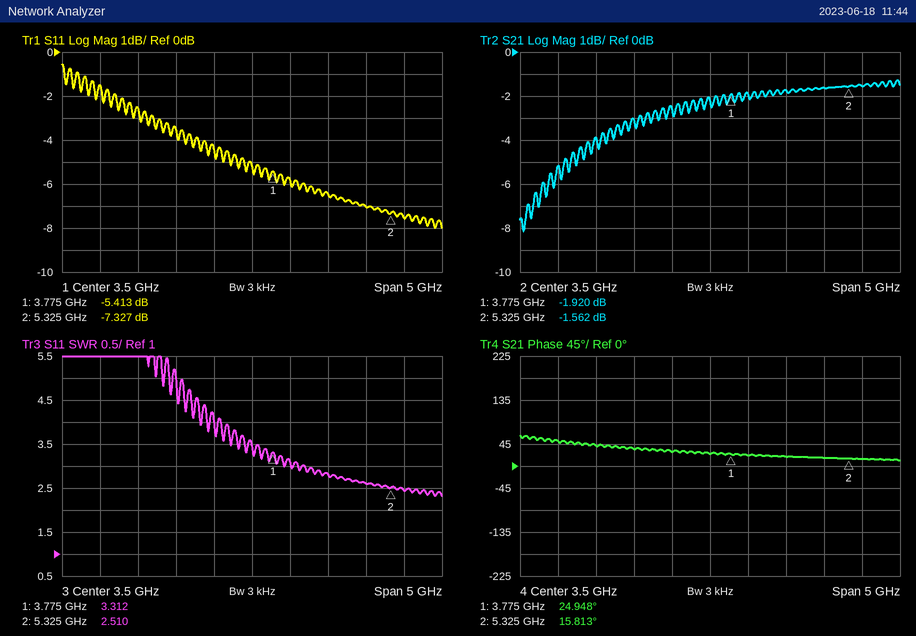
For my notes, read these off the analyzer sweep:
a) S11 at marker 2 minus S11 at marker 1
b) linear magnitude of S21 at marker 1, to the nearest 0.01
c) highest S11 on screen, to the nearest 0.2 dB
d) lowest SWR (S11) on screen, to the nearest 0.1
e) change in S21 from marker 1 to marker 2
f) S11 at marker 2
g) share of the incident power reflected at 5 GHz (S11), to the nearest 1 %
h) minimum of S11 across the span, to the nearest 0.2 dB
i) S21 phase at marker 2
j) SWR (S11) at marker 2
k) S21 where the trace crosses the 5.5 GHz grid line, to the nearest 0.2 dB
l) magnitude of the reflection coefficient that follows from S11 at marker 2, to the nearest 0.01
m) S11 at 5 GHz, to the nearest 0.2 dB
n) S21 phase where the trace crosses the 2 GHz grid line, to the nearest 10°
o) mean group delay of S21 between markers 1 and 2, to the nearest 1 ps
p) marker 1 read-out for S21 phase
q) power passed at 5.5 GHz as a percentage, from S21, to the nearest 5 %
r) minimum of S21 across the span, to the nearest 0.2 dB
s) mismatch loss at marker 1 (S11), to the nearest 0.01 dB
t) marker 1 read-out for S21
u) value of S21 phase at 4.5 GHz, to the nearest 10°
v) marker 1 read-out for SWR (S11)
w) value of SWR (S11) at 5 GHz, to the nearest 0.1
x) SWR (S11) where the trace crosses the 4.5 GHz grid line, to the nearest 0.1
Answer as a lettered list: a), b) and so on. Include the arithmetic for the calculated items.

a) -7.327 − (-5.413) = -1.914 dB
b) 10^(-1.92/20) ≈ 0.80
c) -0.6 dB
d) 2.3
e) -1.562 − (-1.92) = 0.358 dB
f) -7.327 dB
g) 10^(-7/10) ≈ 20 %
h) -8.0 dB
i) 15.813°
j) 2.510
k) -1.6 dB
l) 10^(-7.327/20) ≈ 0.43
m) -7.0 dB
n) 40°
o) −(15.813° − (24.948°))/(360° × 1.55 GHz) ≈ 16 ps
p) 24.948°
q) 10^(-1.6/10) ≈ 69.2 %, so 70 % to the nearest 5 %
r) -8.2 dB
s) −10 log10(1 − 10^(-5.413/10)) ≈ 1.47 dB
t) -1.920 dB
u) 20°
v) 3.312
w) 2.6
x) 2.8
